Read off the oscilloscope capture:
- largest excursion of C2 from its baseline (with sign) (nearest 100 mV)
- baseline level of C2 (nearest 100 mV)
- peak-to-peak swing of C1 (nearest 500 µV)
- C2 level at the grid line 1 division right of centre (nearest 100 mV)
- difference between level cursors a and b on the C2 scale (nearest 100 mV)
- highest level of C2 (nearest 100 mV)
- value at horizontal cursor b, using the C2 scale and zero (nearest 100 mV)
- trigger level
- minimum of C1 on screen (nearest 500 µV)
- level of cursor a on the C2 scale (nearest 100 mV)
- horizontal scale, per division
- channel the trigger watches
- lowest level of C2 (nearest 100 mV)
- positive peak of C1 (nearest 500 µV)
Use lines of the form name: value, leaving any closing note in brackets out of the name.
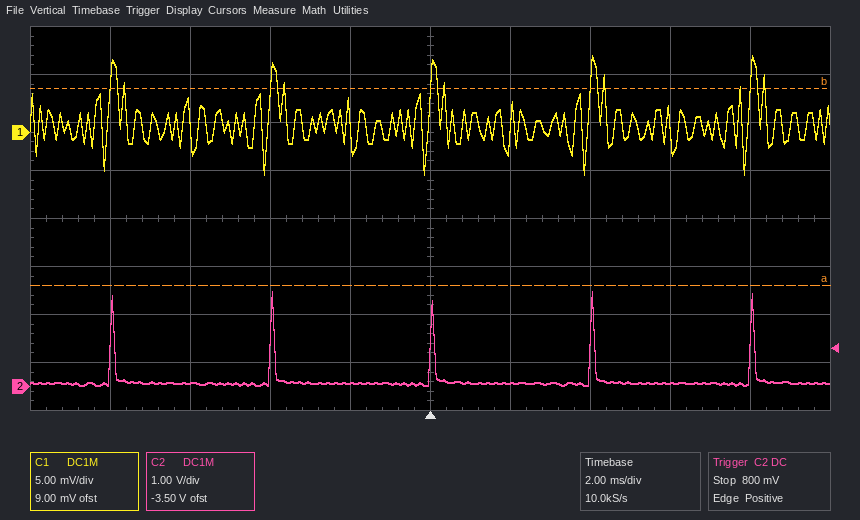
largest excursion of C2 from its baseline (with sign): +1.9 V
baseline level of C2: 100 mV
peak-to-peak swing of C1: 12.5 mV
C2 level at the grid line 1 division right of centre: 100 mV
difference between level cursors a and b on the C2 scale: 4.1 V
highest level of C2: 2.0 V
value at horizontal cursor b, using the C2 scale and zero: 6.2 V
trigger level: 800 mV
minimum of C1 on screen: -4.5 mV
level of cursor a on the C2 scale: 2.1 V
horizontal scale, per division: 2 ms
channel the trigger watches: C2
lowest level of C2: 0.0 V
positive peak of C1: 8.0 mV
